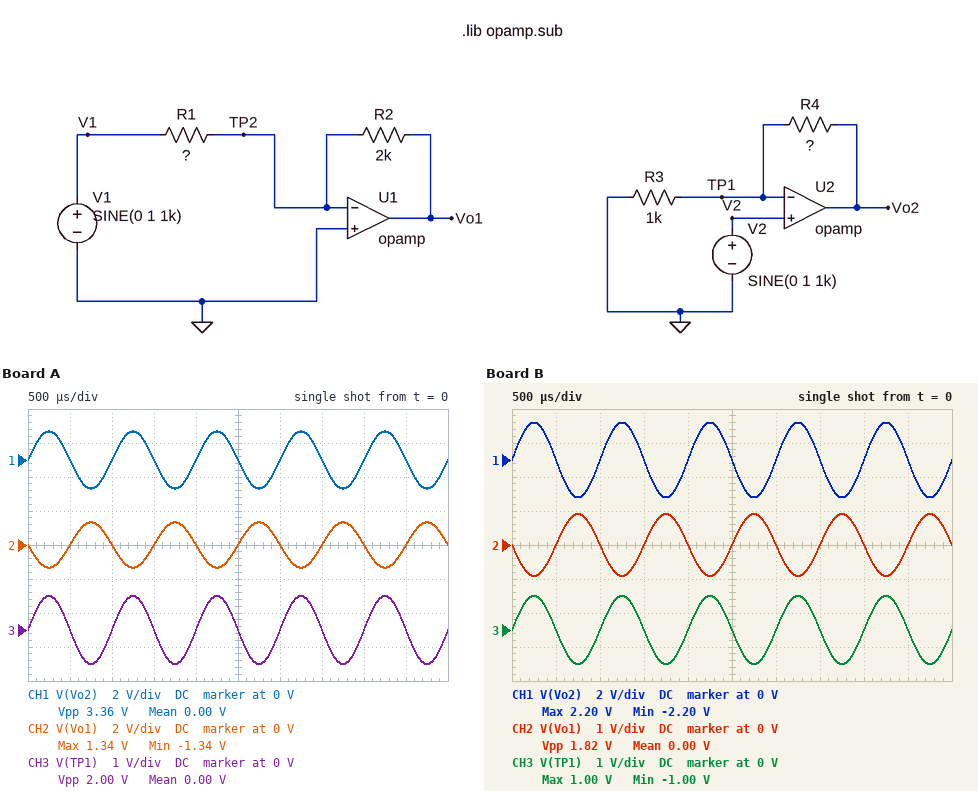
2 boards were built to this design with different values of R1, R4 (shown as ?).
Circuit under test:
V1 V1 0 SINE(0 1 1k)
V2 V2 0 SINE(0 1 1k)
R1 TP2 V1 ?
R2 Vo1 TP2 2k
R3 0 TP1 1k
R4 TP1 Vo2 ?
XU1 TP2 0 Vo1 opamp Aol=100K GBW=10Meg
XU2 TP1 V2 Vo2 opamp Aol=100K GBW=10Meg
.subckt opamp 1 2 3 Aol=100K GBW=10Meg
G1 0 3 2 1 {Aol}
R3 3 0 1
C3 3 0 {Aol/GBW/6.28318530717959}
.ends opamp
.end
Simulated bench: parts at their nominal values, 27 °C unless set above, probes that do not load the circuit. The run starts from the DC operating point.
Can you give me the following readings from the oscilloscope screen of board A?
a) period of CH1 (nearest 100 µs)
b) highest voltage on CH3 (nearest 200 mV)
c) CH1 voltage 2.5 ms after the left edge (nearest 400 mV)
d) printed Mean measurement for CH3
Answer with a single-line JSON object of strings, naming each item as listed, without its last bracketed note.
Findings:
{"period of CH1": "1.0 ms", "highest voltage on CH3": "1.0 V", "CH1 voltage 2.5 ms after the left edge": "0 V", "printed Mean measurement for CH3": "0.00 V"}
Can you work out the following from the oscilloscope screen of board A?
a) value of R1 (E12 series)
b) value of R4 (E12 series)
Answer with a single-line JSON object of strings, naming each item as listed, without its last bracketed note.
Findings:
{"value of R1": "1.5 kΩ", "value of R4": "680 Ω"}
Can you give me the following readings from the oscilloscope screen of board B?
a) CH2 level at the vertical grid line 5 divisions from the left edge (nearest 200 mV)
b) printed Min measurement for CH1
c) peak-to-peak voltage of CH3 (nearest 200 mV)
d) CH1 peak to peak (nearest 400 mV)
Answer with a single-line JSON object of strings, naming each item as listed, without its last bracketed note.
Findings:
{"CH2 level at the vertical grid line 5 divisions from the left edge": "0 V", "printed Min measurement for CH1": "-2.20 V", "peak-to-peak voltage of CH3": "2.0 V", "CH1 peak to peak": "4.4 V"}
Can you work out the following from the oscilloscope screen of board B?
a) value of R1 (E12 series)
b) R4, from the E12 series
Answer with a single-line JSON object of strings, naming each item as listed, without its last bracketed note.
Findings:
{"value of R1": "2.2 kΩ", "R4, from the E12 series": "1.2 kΩ"}
